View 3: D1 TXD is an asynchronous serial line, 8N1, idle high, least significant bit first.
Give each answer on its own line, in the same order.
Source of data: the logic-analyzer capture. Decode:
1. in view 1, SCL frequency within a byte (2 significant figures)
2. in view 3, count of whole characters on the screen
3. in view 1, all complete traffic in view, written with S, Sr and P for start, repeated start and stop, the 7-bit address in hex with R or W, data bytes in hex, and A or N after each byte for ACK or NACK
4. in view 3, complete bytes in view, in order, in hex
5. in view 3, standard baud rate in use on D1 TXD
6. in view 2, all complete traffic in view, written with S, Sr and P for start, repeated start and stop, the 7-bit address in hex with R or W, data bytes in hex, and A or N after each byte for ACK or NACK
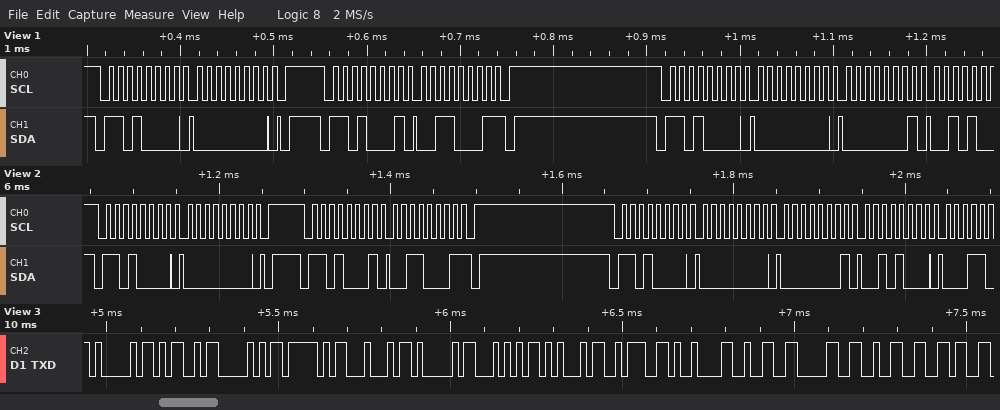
100 kHz
14
S 68W A 00 A P S 68R A 31 N P S 68W A 00 A 01 A
41 4D 50 5F 44 41 54 45 3A 09 32 30 32 36
57600 baud
S 68W A 00 A P S 68R A 31 N P S 68W A 00 A 01 A 28 A
